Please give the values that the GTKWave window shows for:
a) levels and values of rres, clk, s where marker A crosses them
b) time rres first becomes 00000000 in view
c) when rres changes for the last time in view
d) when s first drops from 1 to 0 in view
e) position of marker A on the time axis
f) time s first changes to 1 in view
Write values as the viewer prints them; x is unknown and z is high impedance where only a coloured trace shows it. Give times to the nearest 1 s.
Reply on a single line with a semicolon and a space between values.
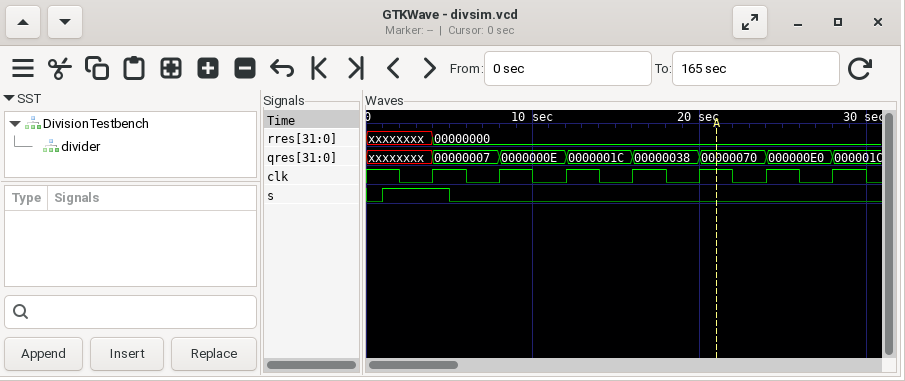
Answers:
rres=00000000, clk=1, s=0; 4 s; 4 s; 5 s; 21 s; 1 s
